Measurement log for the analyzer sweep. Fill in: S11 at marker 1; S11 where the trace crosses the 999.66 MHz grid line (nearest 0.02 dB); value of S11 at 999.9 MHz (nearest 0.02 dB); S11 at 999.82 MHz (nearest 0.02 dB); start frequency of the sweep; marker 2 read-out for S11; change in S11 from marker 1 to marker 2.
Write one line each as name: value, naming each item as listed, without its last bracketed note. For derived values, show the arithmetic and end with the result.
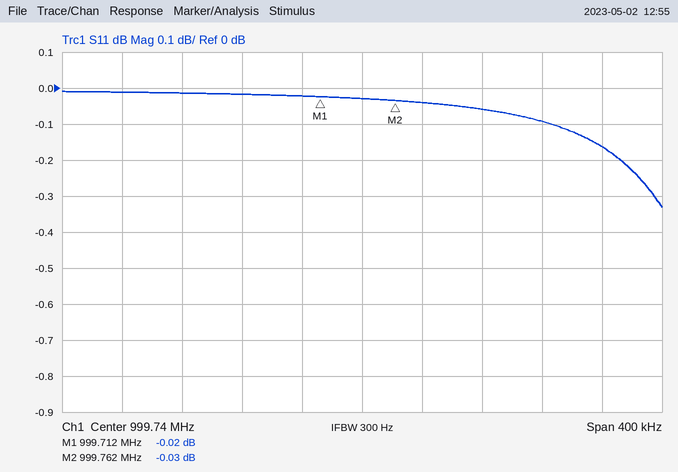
S11 at marker 1: -0.02 dB
S11 where the trace crosses the 999.66 MHz grid line: -0.02 dB
value of S11 at 999.9 MHz: -0.16 dB
S11 at 999.82 MHz: -0.06 dB
start frequency of the sweep: 999.54 MHz
marker 2 read-out for S11: -0.03 dB
change in S11 from marker 1 to marker 2: -0.03 − (-0.02) = -0.01 dB
